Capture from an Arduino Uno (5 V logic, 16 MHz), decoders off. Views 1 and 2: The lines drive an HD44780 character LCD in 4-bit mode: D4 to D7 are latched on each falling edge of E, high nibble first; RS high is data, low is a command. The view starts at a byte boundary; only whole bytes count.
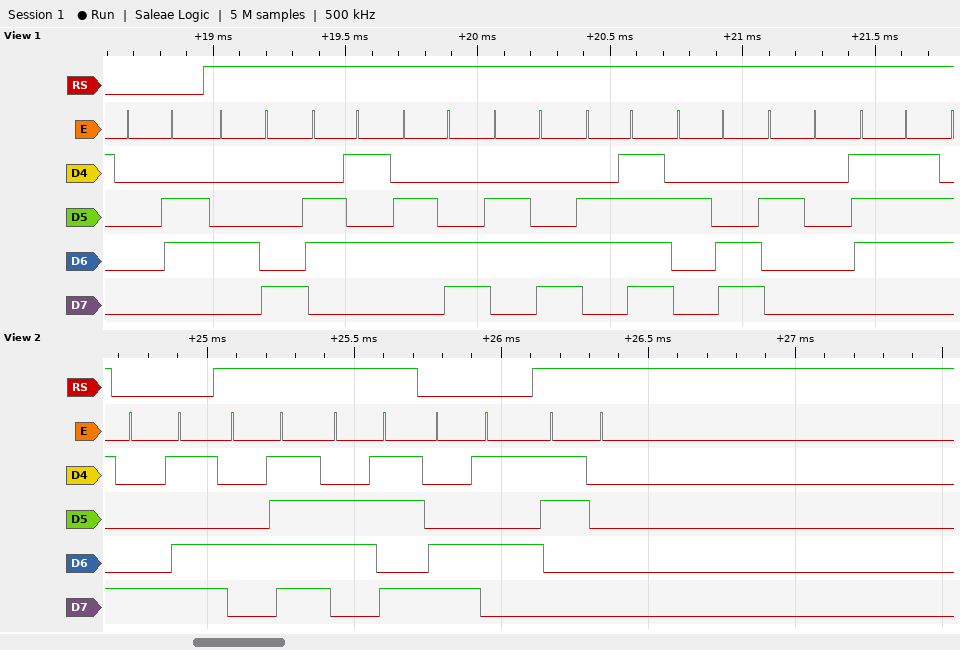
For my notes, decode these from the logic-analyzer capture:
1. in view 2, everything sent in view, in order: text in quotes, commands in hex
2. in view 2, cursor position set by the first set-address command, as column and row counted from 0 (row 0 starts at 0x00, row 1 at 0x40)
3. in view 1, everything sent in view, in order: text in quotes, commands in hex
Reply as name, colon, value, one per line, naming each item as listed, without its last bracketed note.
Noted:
in view 2, everything sent in view, in order: text in quotes, commands in hex: 0x8D "Ok" 0xC5 "0"
in view 2, cursor position set by the first set-address command, as column and row counted from 0: column 13, row 0
in view 1, everything sent in view, in order: text in quotes, commands in hex: 0x06 "Hello, w"
